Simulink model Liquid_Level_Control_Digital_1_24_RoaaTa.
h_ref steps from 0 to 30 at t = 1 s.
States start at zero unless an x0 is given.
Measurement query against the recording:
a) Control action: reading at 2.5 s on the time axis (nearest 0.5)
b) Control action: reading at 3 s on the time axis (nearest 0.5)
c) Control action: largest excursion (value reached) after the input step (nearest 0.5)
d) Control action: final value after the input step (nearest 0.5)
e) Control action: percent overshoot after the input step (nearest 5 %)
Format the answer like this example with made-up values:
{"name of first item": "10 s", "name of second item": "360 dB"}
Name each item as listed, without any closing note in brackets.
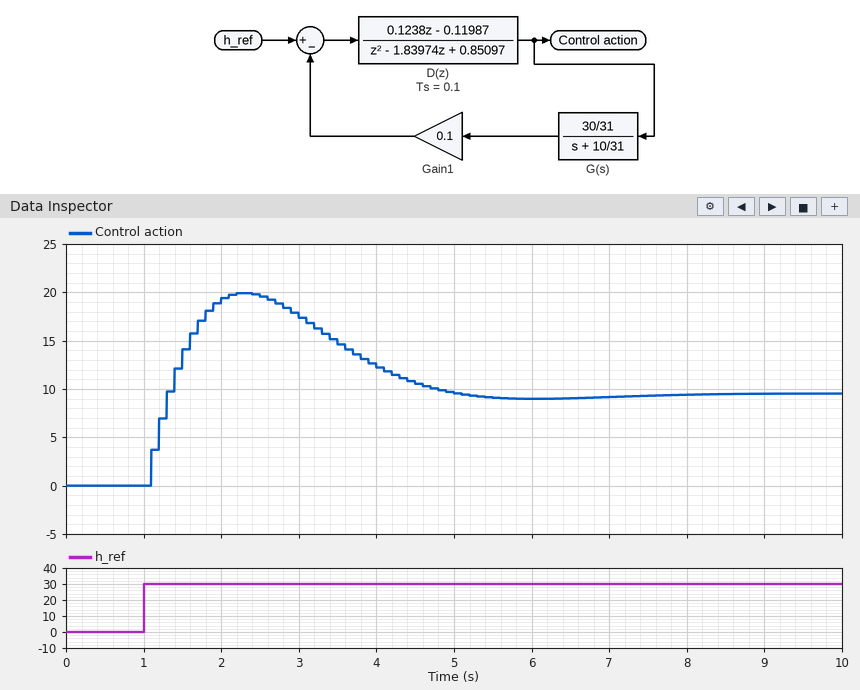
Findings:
{"Control action: reading at 2.5 s on the time axis": "19.5", "Control action: reading at 3 s on the time axis": "17.5", "Control action: largest excursion (value reached) after the input step": "20.0", "Control action: final value after the input step": "9.5", "Control action: percent overshoot after the input step": "110 %"}
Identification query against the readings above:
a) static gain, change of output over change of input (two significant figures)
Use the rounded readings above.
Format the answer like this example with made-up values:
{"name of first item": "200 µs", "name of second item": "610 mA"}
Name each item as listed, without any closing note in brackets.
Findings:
{"static gain, change of output over change of input": "0.32"}
